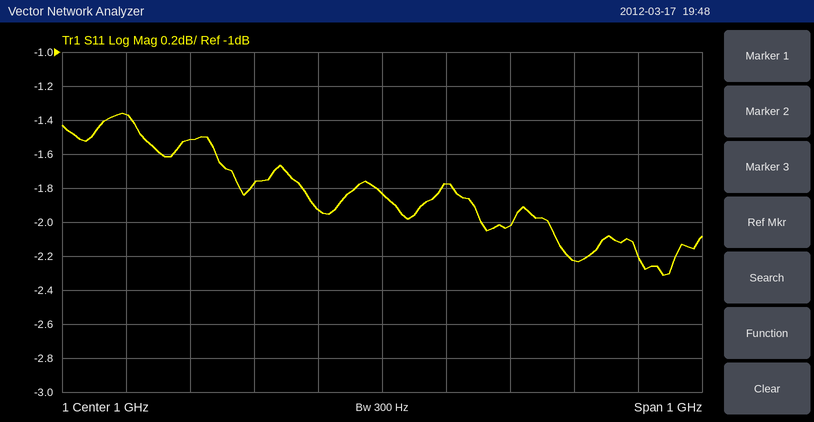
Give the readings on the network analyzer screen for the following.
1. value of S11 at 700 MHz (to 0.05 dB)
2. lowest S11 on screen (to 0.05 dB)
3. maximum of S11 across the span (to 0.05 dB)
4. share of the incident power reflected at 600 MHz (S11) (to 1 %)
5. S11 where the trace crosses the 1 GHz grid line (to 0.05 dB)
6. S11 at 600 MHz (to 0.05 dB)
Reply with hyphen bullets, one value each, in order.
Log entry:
- -1.50 dB
- -2.30 dB
- -1.35 dB
- 73 %
- -1.85 dB
- -1.35 dB
